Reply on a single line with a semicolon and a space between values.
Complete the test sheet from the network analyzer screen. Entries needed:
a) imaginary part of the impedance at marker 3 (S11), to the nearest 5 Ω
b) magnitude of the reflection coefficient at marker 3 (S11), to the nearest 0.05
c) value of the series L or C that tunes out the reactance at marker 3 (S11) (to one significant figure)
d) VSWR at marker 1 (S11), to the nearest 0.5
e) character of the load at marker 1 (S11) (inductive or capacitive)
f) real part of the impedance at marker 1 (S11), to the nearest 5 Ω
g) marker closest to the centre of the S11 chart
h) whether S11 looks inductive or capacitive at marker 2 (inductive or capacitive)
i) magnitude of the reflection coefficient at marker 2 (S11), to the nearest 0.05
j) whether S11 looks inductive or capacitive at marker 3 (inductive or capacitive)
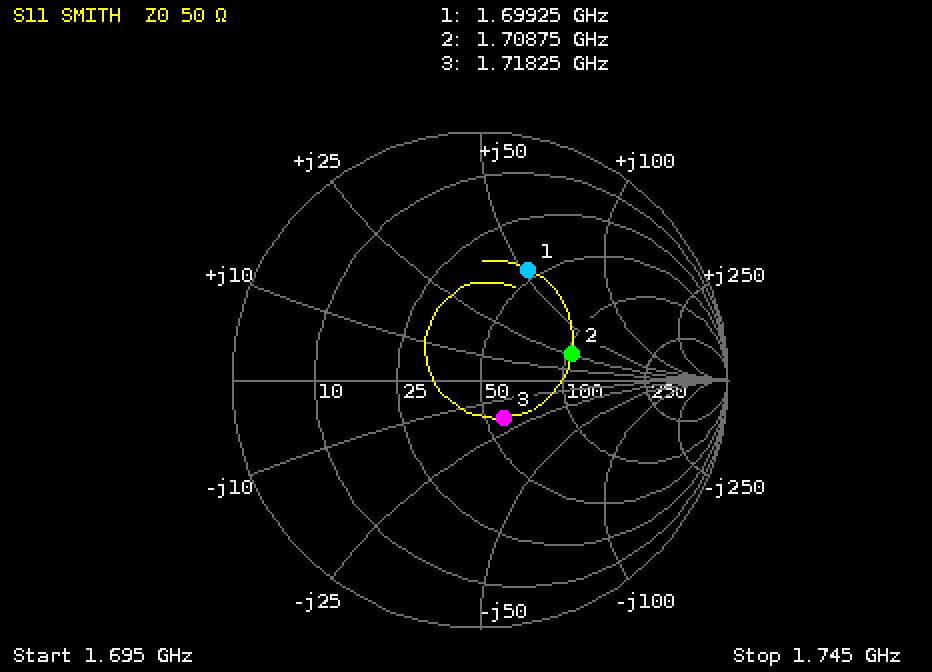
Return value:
-20 Ω; 0.20; 2 nH; 3.0; inductive; 45 Ω; marker 3; inductive; 0.40; capacitive
